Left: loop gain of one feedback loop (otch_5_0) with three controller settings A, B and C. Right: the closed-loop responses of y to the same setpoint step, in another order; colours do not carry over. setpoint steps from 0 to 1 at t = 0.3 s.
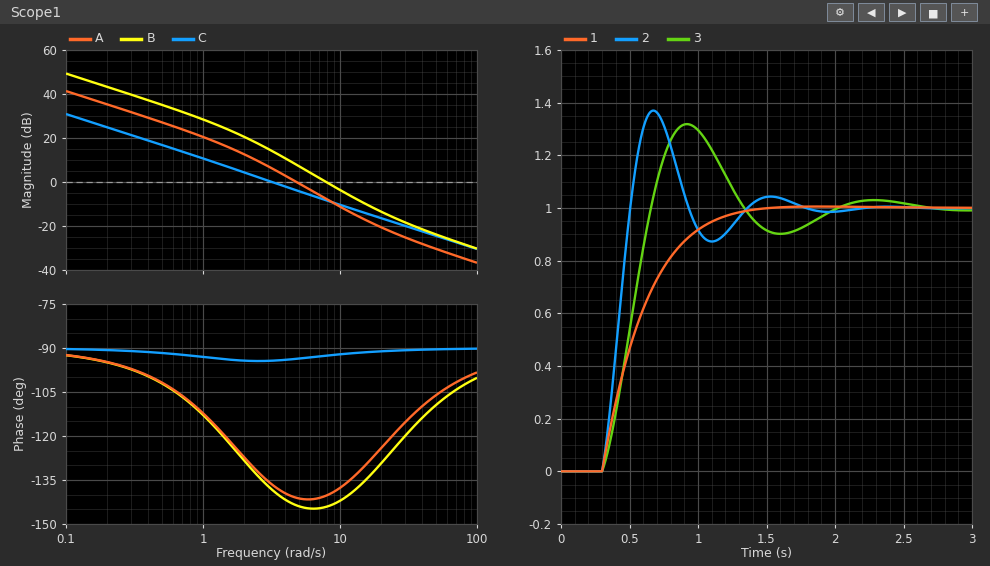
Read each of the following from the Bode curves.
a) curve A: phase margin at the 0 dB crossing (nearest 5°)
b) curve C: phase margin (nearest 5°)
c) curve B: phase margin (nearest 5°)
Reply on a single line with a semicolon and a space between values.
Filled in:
40°; 85°; 35°
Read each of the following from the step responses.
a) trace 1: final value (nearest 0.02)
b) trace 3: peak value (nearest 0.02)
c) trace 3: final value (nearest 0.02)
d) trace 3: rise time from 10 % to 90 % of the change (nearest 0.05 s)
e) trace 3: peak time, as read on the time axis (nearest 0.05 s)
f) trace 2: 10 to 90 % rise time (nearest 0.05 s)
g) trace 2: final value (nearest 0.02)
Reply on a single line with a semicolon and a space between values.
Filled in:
1.00; 1.32; 1.00; 0.25 s; 0.90 s; 0.15 s; 1.00
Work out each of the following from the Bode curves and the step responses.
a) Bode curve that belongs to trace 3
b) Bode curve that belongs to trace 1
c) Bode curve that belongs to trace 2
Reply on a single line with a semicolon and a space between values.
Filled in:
A; C; B
